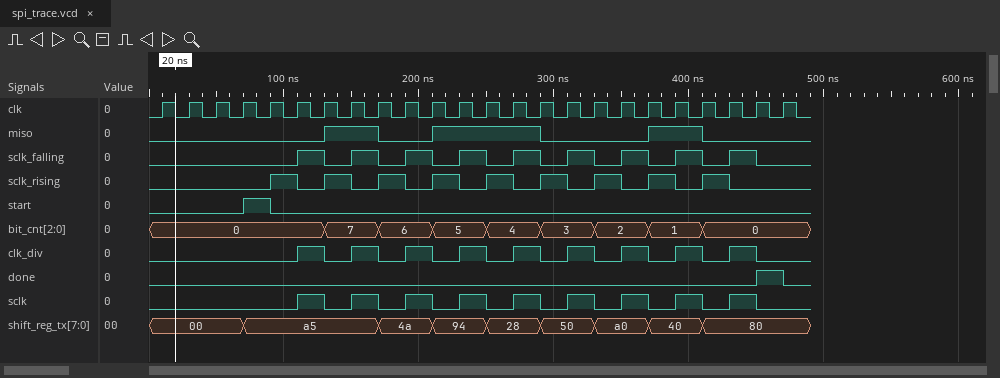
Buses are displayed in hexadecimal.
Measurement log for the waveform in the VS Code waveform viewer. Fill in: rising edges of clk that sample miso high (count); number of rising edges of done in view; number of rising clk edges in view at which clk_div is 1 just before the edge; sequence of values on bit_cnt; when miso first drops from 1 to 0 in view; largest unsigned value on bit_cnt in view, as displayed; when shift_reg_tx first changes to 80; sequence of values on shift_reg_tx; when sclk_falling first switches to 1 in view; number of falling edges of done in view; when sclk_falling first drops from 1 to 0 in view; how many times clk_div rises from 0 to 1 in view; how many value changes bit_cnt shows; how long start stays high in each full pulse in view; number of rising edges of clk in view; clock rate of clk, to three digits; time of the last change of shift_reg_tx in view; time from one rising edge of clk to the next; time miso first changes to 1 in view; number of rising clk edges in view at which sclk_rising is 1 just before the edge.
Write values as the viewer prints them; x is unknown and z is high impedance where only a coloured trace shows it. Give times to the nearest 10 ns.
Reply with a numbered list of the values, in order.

1. 8
2. 1
3. 9
4. 0, 7, 6, 5, 4, 3, 2, 1, 0
5. 170 ns
6. 7
7. 410 ns
8. 00, a5, 4a, 94, 28, 50, a0, 40, 80
9. 110 ns
10. 1
11. 130 ns
12. 9
13. 8
14. 20 ns
15. 24
16. 50.0 MHz
17. 410 ns
18. 20 ns
19. 130 ns
20. 9
